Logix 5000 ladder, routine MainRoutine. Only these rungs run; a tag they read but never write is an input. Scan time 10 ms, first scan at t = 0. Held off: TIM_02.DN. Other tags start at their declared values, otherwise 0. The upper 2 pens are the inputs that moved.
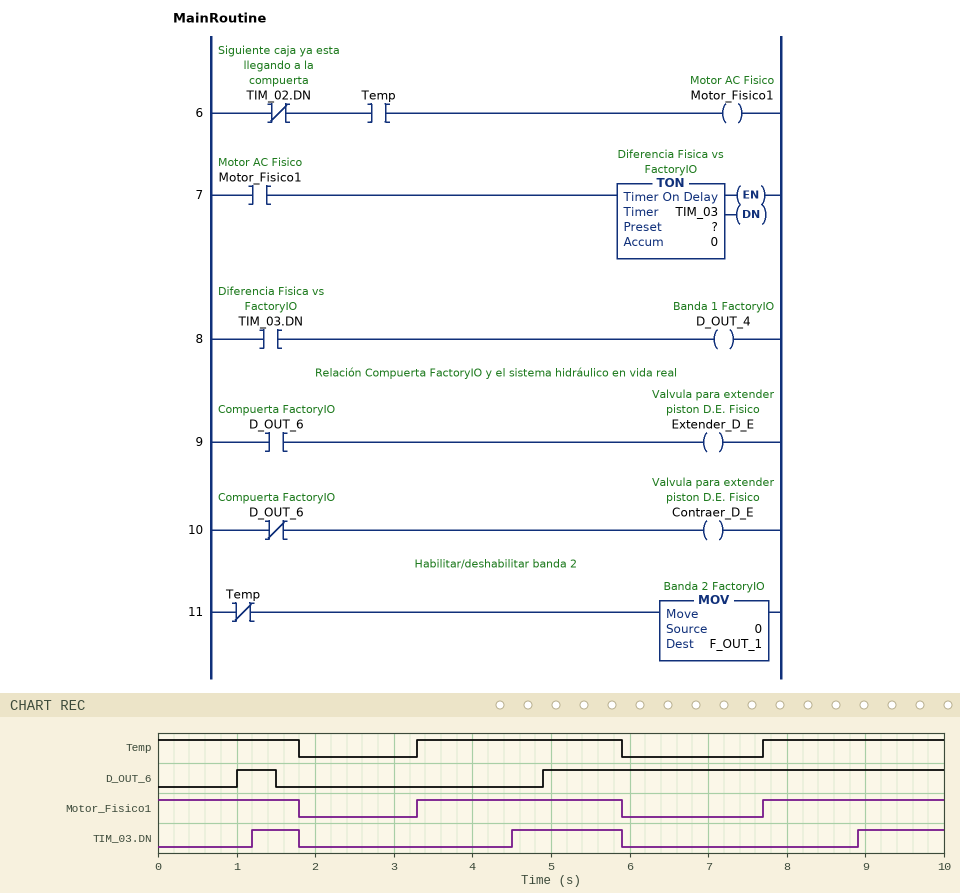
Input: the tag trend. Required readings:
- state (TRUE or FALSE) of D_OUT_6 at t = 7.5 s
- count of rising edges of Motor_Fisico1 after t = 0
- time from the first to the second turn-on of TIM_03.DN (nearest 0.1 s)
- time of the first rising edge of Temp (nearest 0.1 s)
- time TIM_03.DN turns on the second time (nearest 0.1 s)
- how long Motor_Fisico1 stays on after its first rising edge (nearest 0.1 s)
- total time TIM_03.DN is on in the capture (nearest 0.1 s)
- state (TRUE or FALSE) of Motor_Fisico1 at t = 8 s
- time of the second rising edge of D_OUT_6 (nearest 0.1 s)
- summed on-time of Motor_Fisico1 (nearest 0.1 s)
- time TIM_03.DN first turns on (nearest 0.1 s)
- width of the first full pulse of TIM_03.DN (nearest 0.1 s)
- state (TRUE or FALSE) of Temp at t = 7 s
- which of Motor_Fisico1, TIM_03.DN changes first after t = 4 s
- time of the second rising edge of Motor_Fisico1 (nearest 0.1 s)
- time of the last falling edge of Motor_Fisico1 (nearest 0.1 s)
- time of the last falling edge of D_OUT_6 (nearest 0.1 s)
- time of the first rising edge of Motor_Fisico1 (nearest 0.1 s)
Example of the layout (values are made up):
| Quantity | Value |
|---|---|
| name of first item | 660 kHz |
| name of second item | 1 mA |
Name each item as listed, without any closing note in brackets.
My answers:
| Quantity | Value |
|---|---|
| state (TRUE or FALSE) of D_OUT_6 at t = 7.5 s | TRUE |
| count of rising edges of Motor_Fisico1 after t = 0 | 2 |
| time from the first to the second turn-on of TIM_03.DN | 3.3 s |
| time of the first rising edge of Temp | 3.3 s |
| time TIM_03.DN turns on the second time | 4.5 s |
| how long Motor_Fisico1 stays on after its first rising edge | 2.6 s |
| total time TIM_03.DN is on in the capture | 3.1 s |
| state (TRUE or FALSE) of Motor_Fisico1 at t = 8 s | TRUE |
| time of the second rising edge of D_OUT_6 | 4.9 s |
| summed on-time of Motor_Fisico1 | 6.7 s |
| time TIM_03.DN first turns on | 1.2 s |
| width of the first full pulse of TIM_03.DN | 0.6 s |
| state (TRUE or FALSE) of Temp at t = 7 s | FALSE |
| which of Motor_Fisico1, TIM_03.DN changes first after t = 4 s | TIM_03.DN |
| time of the second rising edge of Motor_Fisico1 | 7.7 s |
| time of the last falling edge of Motor_Fisico1 | 5.9 s |
| time of the last falling edge of D_OUT_6 | 1.5 s |
| time of the first rising edge of Motor_Fisico1 | 3.3 s |
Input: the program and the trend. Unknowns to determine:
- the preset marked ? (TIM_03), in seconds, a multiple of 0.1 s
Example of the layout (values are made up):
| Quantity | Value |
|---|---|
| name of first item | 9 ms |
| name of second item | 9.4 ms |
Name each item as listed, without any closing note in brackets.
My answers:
| Quantity | Value |
|---|---|
| the preset marked ? (TIM_03), in seconds, a multiple of 0.1 s | 1.2 s |
